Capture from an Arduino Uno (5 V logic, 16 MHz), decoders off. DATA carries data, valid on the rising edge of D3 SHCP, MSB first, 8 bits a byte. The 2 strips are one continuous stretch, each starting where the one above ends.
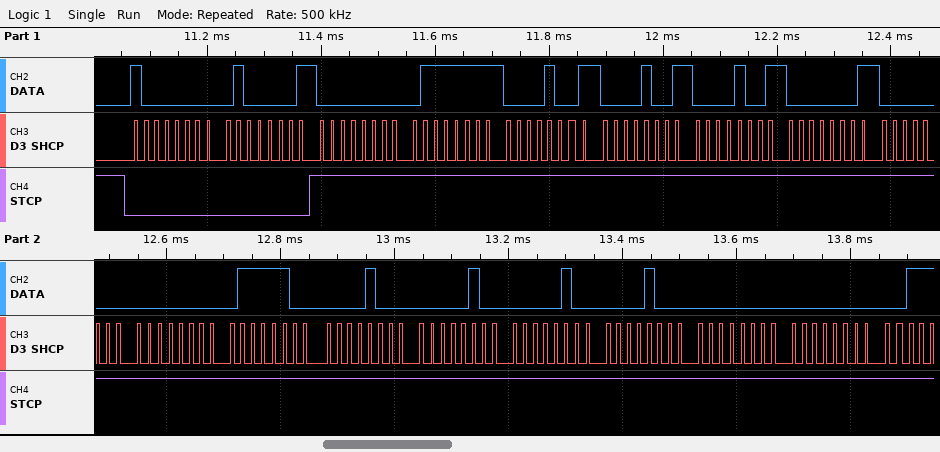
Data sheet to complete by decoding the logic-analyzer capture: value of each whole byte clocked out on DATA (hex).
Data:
80 41 00 7F 09 09 09 01 00 00 7C 08 04 04 08 00 00
